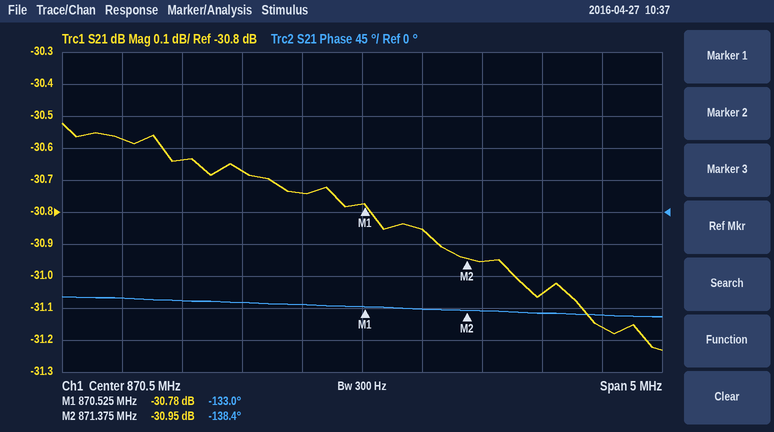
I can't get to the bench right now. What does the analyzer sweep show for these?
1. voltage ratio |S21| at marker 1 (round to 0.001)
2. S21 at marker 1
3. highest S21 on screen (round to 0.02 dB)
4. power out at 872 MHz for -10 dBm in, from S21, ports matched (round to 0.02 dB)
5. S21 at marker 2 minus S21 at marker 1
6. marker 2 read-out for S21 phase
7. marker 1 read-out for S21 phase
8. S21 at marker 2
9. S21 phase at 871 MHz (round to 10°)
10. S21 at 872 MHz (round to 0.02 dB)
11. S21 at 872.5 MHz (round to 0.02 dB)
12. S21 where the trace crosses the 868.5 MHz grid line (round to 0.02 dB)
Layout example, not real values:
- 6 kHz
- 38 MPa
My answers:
- 0.029
- -30.78 dB
- -30.52 dB
- -41.06 dBm
- -0.17 dB
- -138.4°
- -133.0°
- -30.95 dB
- -140°
- -31.06 dB
- -31.16 dB
- -30.58 dB
